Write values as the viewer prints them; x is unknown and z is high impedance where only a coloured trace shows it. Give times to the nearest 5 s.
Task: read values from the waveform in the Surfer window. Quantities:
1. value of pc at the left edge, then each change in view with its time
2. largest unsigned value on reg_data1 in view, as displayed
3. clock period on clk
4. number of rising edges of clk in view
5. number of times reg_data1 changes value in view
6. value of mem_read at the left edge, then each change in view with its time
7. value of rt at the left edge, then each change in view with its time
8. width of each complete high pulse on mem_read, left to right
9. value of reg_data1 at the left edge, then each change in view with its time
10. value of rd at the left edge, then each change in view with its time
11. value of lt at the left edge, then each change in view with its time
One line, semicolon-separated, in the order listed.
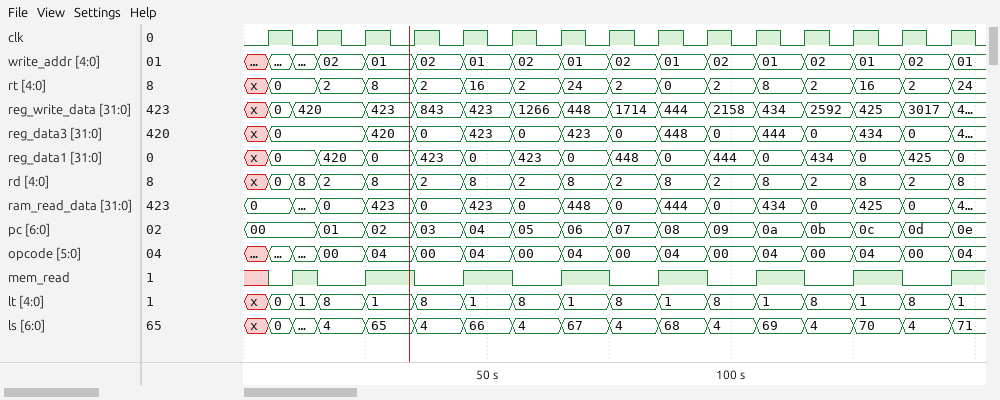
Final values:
00, 01 at 15 s, 02 at 25 s, 03 at 35 s, 04 at 45 s, 05 at 55 s, 06 at 65 s, 07 at 75 s, 08 at 85 s, 09 at 95 s, 0a at 105 s, 0b at 115 s, 0c at 125 s, 0d at 135 s, 0e at 145 s; 448; 10 s; 15; 15; x, 0 at 5 s, 1 at 10 s, 0 at 15 s, 1 at 25 s, 0 at 35 s, 1 at 45 s, 0 at 55 s, 1 at 65 s, 0 at 75 s, 1 at 85 s, 0 at 95 s, 1 at 105 s, 0 at 115 s, 1 at 125 s, 0 at 135 s, 1 at 145 s; x, 0 at 5 s, 2 at 15 s, 8 at 25 s, 2 at 35 s, 16 at 45 s, 2 at 55 s, 24 at 65 s, 2 at 75 s, 0 at 85 s, 2 at 95 s, 8 at 105 s, 2 at 115 s, 16 at 125 s, 2 at 135 s, 24 at 145 s; 5 s, 10 s, 10 s, 10 s, 10 s, 10 s, 10 s; x, 0 at 5 s, 420 at 15 s, 0 at 25 s, 423 at 35 s, 0 at 45 s, 423 at 55 s, 0 at 65 s, 448 at 75 s, 0 at 85 s, 444 at 95 s, 0 at 105 s, 434 at 115 s, 0 at 125 s, 425 at 135 s, 0 at 145 s; x, 0 at 5 s, 8 at 10 s, 2 at 15 s, 8 at 25 s, 2 at 35 s, 8 at 45 s, 2 at 55 s, 8 at 65 s, 2 at 75 s, 8 at 85 s, 2 at 95 s, 8 at 105 s, 2 at 115 s, 8 at 125 s, 2 at 135 s, 8 at 145 s; x, 0 at 5 s, 1 at 10 s, 8 at 15 s, 1 at 25 s, 8 at 35 s, 1 at 45 s, 8 at 55 s, 1 at 65 s, 8 at 75 s, 1 at 85 s, 8 at 95 s, 1 at 105 s, 8 at 115 s, 1 at 125 s, 8 at 135 s, 1 at 145 s
